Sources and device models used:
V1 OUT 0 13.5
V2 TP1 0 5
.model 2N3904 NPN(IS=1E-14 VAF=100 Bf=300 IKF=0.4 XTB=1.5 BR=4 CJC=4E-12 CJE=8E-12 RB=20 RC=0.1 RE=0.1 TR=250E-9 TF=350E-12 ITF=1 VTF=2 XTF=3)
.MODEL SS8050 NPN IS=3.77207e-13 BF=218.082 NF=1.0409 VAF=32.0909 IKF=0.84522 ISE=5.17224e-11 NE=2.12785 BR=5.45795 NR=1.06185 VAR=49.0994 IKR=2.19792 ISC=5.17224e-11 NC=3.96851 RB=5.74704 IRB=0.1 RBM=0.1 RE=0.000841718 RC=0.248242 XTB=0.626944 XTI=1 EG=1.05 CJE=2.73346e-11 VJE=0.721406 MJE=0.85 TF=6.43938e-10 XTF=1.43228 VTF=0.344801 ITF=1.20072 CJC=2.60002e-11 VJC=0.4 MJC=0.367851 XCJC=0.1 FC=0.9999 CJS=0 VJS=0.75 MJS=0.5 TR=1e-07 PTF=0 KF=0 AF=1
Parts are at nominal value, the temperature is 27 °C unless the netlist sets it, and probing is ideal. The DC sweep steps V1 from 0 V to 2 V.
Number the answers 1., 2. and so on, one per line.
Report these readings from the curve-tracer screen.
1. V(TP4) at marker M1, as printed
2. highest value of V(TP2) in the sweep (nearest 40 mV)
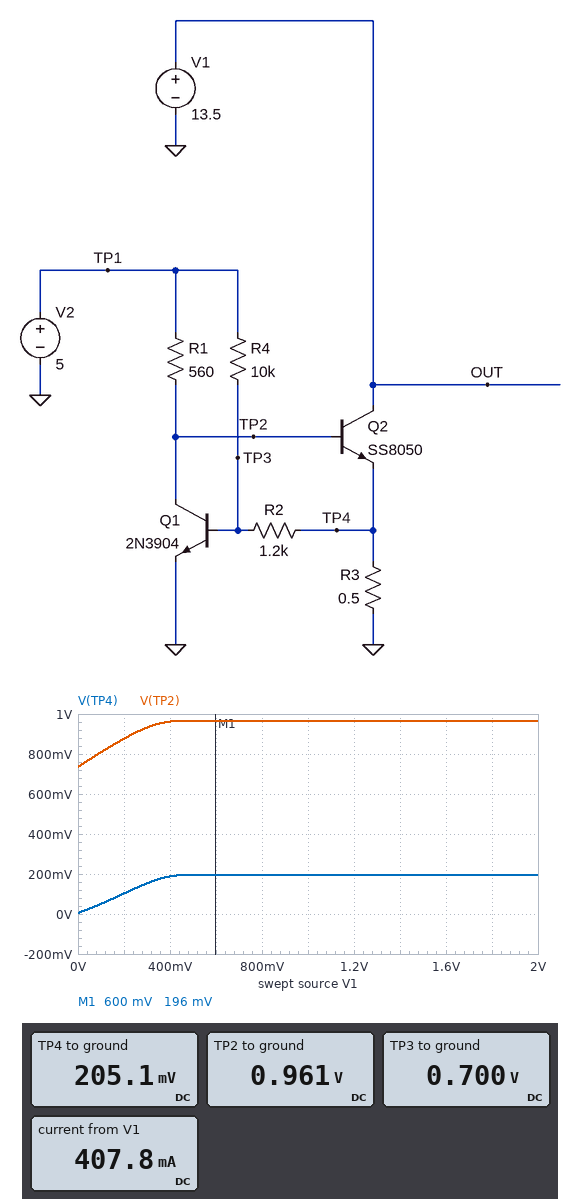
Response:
1. 196 mV
2. 960 mV
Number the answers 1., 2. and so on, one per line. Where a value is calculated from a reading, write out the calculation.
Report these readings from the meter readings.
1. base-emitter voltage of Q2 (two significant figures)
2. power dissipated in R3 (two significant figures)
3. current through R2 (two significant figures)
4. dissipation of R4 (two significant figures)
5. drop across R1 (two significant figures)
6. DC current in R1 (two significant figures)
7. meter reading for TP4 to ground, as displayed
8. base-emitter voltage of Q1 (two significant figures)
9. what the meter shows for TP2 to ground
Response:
1. 961 mV - 205.1 mV = 760 mV
2. (205.1 mV)^2 / 500 mΩ = 84 mW
3. (700 mV - 205.1 mV) / 1.2 kΩ = 410 µA
4. (5 V - 700 mV)^2 / 10 kΩ = 1.8 mW
5. 5 V - 961 mV = 4.0 V
6. (5 V - 961 mV) / 560 Ω = 7.2 mA
7. 205.1 mV
8. 700 mV = 700 mV
9. 0.961 V
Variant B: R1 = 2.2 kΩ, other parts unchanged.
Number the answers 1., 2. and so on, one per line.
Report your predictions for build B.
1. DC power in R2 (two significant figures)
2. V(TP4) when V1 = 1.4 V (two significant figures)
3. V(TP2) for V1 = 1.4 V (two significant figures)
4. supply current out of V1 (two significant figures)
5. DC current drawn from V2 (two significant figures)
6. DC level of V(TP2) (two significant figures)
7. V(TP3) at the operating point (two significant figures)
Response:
1. 220 µW
2. 120 mV
3. 860 mV
4. 260 mA
5. 2.3 mA
6. 870 mV
7. 650 mV
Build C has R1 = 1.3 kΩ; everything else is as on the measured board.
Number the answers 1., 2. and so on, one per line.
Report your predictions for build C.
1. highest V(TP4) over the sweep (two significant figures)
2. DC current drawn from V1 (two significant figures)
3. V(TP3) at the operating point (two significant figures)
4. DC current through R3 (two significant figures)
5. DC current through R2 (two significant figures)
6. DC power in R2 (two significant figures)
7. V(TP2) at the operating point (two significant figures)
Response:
1. 150 mV
2. 310 mA
3. 670 mV
4. 320 mA
5. 430 µA
6. 220 µW
7. 900 mV
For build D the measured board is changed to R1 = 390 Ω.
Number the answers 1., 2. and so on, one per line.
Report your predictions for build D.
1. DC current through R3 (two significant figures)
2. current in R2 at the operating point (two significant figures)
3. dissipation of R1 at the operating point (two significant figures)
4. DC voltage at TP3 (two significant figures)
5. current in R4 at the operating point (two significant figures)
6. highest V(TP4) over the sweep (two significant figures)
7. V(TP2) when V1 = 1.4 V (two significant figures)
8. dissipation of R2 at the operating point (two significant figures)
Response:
1. 460 mA
2. 400 µA
3. 41 mW
4. 710 mV
5. 430 µA
6. 220 mV
7. 1.0 V
8. 190 µW
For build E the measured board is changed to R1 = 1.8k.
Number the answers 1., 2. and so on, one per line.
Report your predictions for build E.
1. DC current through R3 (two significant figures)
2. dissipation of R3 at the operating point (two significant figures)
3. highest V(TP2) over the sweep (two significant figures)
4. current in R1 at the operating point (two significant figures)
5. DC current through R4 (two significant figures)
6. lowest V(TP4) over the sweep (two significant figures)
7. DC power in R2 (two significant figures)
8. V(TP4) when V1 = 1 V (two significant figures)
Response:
1. 280 mA
2. 40 mW
3. 880 mV
4. 2.3 mA
5. 430 µA
6. 2.8 mV
7. 220 µW
8. 130 mV
